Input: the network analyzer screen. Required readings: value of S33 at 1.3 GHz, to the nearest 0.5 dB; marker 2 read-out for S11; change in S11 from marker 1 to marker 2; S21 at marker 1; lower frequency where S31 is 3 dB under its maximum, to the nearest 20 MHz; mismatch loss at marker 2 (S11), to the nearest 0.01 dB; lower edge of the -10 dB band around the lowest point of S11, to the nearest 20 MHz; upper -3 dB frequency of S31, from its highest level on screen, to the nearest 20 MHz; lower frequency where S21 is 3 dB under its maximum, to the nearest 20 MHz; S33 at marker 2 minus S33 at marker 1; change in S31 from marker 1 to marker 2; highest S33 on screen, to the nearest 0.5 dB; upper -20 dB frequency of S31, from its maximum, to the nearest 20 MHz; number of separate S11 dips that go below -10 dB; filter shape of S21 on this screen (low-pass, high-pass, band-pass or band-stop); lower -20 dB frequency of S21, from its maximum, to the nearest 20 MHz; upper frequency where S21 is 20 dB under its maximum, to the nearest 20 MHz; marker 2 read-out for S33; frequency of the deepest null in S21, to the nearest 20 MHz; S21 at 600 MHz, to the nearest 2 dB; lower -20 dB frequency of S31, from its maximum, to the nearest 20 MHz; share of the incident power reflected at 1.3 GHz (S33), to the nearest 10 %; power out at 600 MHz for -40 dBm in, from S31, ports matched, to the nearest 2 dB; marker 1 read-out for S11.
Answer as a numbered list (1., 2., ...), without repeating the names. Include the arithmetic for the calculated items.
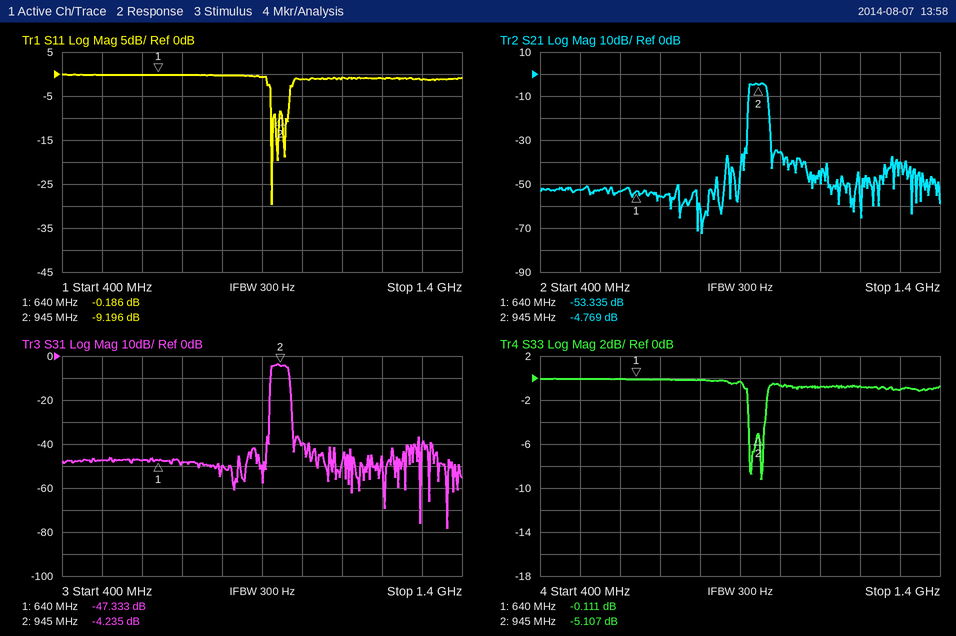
1. -1.0 dB
2. -9.196 dB
3. -9.196 − (-0.186) = -9.010 dB
4. -53.335 dB
5. 920 MHz
6. −10 log10(1 − 10^(-9.196/10)) ≈ 0.56 dB
7. 920 MHz
8. 960 MHz
9. 920 MHz
10. -5.107 − (-0.111) = -4.996 dB
11. -4.235 − (-47.333) = 43.098 dB
12. 0.0 dB
13. 980 MHz
14. 3
15. band-pass
16. 920 MHz
17. 980 MHz
18. -5.107 dB
19. 800 MHz
20. -54 dB
21. 920 MHz
22. 10^(-1/10) ≈ 79.4 %, so 80 % to the nearest 10 %
23. -40 dBm + (-48 dB) = -88 dBm
24. -0.186 dB
